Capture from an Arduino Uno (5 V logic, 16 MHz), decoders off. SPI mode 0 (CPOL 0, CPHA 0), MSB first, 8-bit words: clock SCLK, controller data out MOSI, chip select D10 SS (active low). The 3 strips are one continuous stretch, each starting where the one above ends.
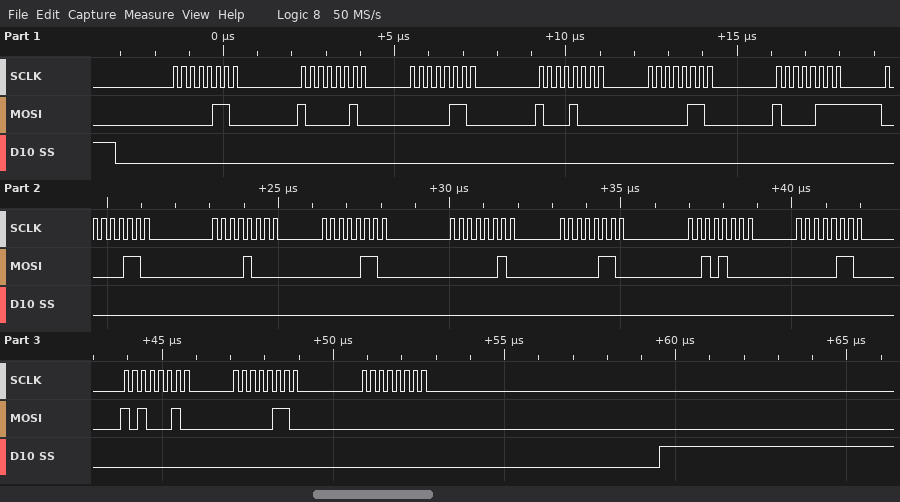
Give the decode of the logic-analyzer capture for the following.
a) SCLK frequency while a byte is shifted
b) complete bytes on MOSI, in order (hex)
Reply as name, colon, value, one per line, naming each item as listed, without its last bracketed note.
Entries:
SCLK frequency while a byte is shifted: 4 MHz
complete bytes on MOSI, in order: 06 82 06 88 06 87 06 08 06 02 06 28 06 A2 06 00
